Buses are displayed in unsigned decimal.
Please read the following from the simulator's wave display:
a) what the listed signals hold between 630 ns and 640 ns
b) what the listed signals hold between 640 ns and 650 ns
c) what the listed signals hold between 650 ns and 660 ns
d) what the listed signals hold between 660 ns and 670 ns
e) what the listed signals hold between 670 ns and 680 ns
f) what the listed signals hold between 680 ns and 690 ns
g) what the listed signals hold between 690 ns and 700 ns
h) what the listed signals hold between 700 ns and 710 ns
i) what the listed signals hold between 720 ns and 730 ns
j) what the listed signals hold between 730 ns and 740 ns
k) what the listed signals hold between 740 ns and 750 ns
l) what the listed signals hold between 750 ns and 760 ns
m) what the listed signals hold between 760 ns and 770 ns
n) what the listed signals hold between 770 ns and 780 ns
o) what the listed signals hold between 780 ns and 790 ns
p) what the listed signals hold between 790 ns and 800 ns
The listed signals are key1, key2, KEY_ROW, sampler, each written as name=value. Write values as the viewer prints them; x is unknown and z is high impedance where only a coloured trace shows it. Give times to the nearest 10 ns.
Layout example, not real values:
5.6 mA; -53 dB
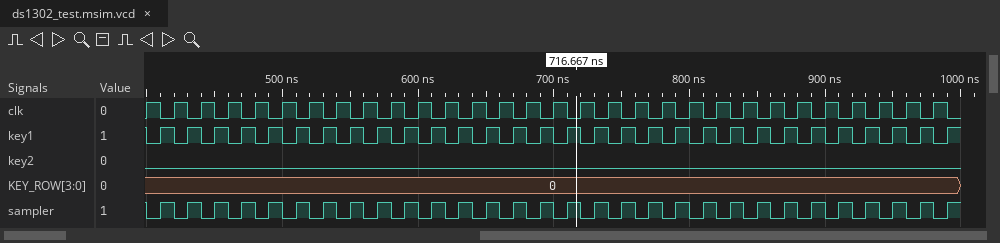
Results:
key1=1, key2=0, KEY_ROW=0, sampler=1; key1=0, key2=0, KEY_ROW=0, sampler=0; key1=1, key2=0, KEY_ROW=0, sampler=1; key1=0, key2=0, KEY_ROW=0, sampler=0; key1=1, key2=0, KEY_ROW=0, sampler=1; key1=0, key2=0, KEY_ROW=0, sampler=0; key1=1, key2=0, KEY_ROW=0, sampler=1; key1=0, key2=0, KEY_ROW=0, sampler=0; key1=0, key2=0, KEY_ROW=0, sampler=0; key1=1, key2=0, KEY_ROW=0, sampler=1; key1=0, key2=0, KEY_ROW=0, sampler=0; key1=1, key2=0, KEY_ROW=0, sampler=1; key1=0, key2=0, KEY_ROW=0, sampler=0; key1=1, key2=0, KEY_ROW=0, sampler=1; key1=0, key2=0, KEY_ROW=0, sampler=0; key1=1, key2=0, KEY_ROW=0, sampler=1
